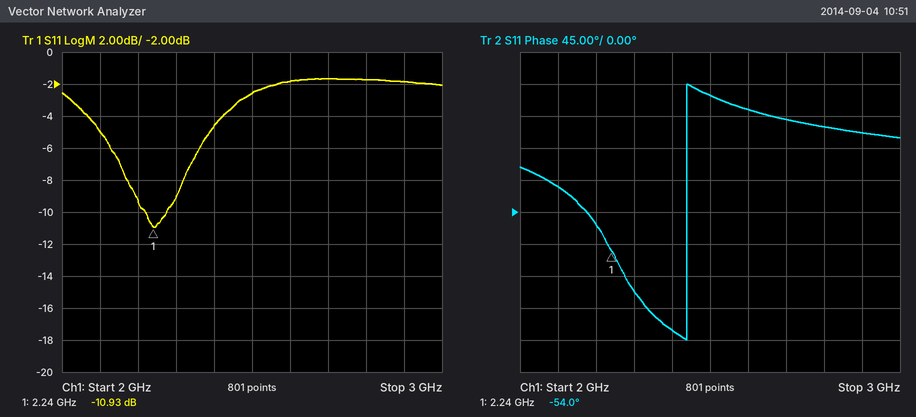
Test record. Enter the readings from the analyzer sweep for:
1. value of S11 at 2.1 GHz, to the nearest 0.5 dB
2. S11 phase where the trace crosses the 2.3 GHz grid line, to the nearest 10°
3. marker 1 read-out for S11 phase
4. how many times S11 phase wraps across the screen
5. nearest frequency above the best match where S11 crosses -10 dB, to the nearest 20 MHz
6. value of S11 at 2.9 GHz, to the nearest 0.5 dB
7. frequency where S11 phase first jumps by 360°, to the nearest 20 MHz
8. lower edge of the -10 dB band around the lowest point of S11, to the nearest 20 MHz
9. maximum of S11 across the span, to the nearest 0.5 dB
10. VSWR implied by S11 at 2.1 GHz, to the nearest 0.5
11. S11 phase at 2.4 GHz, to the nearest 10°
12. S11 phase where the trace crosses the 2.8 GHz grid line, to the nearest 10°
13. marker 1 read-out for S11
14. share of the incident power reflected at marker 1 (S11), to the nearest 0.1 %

-5.0 dB
-110°
-54.0°
1
2.28 GHz
-2.0 dB
2.44 GHz
2.22 GHz
-1.5 dB
3.5
-170°
120°
-10.93 dB
8.1 %
